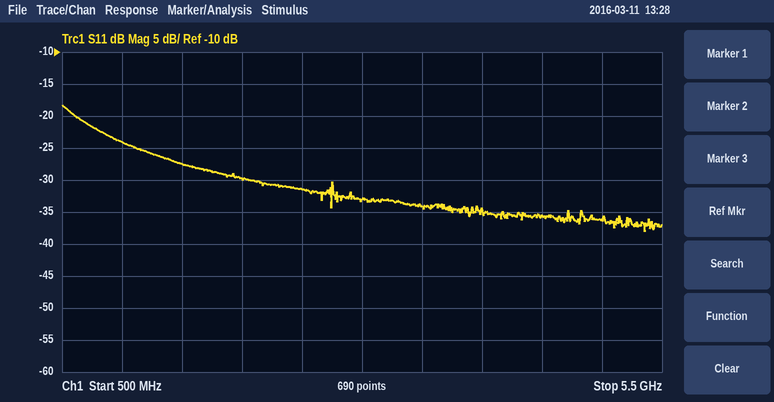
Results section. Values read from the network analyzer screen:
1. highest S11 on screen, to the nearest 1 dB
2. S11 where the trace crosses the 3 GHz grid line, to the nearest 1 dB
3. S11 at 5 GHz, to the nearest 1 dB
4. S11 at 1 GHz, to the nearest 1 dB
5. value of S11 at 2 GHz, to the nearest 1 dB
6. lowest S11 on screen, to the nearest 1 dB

-18 dB
-33 dB
-36 dB
-24 dB
-30 dB
-38 dB
